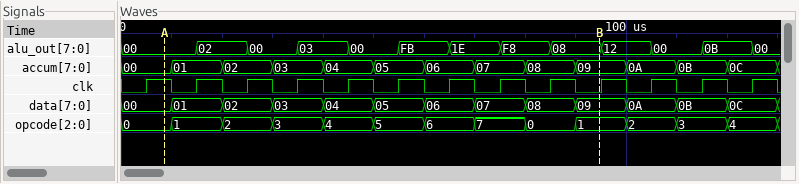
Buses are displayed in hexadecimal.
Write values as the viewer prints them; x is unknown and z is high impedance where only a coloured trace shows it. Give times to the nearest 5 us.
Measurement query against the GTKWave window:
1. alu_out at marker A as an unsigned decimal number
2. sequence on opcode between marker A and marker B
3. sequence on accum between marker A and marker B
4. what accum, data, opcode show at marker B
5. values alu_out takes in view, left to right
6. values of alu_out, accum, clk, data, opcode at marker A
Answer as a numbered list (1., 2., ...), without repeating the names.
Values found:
1. 0
2. 0, 1, 2, 3, 4, 5, 6, 7, 0, 1
3. 00, 01, 02, 03, 04, 05, 06, 07, 08, 09
4. accum=09, data=09, opcode=1
5. 00, 02, 00, 03, 00, FB, 1E, F8, 08, 12, 00, 0B, 00
6. alu_out=00, accum=00, clk=1, data=00, opcode=0
